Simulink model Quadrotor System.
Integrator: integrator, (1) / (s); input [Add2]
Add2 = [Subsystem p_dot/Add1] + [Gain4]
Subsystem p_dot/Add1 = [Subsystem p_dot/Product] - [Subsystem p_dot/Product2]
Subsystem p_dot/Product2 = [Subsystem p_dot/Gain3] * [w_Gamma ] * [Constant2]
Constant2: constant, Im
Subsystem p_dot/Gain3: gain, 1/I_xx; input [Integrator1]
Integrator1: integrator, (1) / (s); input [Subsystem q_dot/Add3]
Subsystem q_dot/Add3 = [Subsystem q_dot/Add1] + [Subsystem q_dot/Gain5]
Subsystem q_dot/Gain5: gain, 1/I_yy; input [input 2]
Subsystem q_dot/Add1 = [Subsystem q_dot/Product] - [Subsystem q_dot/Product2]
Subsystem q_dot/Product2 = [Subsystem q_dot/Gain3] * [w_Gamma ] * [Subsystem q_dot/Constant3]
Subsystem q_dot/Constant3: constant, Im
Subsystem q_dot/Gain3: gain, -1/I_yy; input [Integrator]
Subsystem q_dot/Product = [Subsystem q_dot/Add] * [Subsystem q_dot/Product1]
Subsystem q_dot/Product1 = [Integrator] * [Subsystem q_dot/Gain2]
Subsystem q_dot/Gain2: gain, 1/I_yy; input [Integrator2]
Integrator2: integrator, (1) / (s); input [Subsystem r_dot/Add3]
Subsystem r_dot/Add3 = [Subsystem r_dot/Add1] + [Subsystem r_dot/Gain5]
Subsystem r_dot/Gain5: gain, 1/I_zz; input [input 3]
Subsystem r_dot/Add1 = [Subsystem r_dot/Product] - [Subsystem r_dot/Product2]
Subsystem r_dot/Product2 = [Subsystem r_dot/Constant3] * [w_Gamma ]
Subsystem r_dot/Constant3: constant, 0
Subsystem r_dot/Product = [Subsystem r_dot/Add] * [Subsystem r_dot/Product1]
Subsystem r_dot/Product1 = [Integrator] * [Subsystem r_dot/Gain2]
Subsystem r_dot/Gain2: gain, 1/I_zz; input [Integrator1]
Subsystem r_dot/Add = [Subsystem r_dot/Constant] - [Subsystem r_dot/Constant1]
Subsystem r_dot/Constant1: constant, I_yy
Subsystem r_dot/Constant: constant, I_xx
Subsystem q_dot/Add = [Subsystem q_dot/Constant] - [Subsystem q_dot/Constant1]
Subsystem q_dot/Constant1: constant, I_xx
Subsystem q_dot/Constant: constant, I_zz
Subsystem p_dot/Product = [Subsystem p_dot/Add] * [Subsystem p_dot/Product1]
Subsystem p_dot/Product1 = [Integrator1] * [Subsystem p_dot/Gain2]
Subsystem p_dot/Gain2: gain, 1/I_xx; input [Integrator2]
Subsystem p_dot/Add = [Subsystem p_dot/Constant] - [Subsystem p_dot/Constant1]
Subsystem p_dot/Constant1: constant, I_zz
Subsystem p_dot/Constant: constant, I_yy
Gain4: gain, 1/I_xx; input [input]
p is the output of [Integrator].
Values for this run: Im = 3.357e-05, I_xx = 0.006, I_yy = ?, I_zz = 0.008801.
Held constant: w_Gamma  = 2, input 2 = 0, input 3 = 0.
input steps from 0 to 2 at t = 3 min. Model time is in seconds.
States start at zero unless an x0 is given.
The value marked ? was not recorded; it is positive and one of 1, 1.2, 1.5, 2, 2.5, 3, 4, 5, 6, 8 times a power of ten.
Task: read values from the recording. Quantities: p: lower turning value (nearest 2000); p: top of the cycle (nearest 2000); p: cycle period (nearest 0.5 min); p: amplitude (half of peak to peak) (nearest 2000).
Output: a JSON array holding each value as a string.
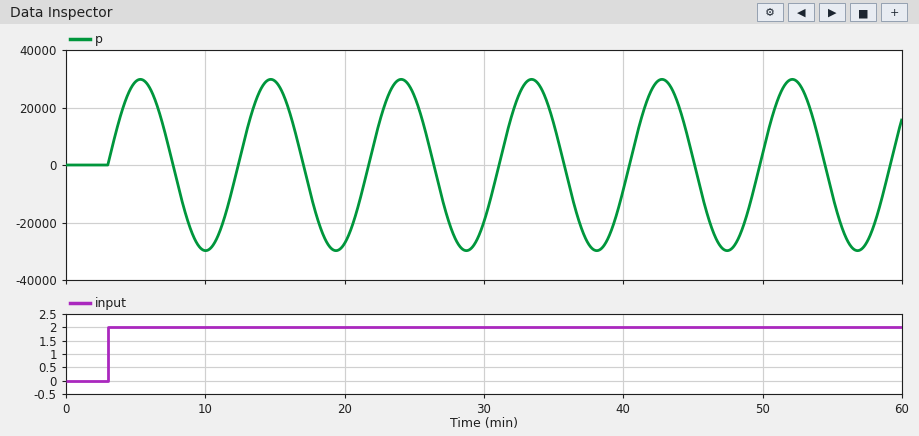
["-30000", "30000", "9.5 min", "30000"]
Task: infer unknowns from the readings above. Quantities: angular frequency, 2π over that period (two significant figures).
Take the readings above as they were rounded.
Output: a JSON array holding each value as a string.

["0.66 rad/min"]
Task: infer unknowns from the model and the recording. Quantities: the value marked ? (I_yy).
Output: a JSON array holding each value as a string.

["0.006"]
